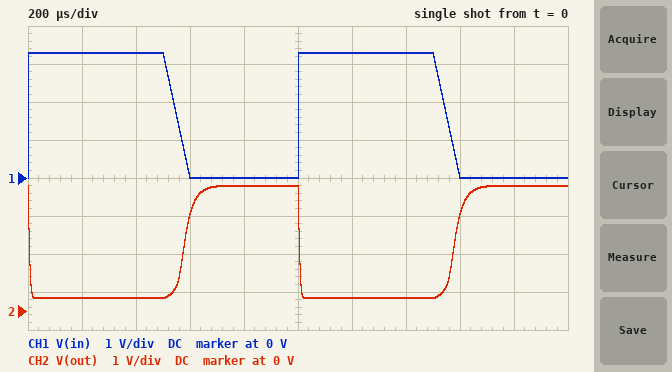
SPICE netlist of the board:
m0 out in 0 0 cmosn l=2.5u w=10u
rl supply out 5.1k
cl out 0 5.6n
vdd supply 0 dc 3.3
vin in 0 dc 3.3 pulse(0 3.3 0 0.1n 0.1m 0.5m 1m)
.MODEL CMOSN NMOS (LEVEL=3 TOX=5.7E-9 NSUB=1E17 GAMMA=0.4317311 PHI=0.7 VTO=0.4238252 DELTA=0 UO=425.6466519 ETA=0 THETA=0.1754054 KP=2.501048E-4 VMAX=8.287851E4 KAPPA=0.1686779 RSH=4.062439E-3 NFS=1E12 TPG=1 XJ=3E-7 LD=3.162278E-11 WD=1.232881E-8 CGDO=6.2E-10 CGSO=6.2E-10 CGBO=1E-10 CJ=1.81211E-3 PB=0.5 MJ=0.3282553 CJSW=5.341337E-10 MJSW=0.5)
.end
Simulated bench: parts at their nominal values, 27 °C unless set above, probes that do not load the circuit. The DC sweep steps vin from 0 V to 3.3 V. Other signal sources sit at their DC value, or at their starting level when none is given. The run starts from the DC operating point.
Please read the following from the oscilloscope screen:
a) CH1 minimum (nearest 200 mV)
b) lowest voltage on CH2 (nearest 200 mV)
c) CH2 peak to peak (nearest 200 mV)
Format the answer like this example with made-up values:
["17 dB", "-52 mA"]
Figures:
["0 V", "400 mV", "3.0 V"]
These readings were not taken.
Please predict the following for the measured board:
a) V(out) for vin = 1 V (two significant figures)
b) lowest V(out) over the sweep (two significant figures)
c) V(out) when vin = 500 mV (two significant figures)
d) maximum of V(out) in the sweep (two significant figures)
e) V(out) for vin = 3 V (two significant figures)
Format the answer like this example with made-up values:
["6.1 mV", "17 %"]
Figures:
["2.6 V", "340 mV", "3.3 V", "3.3 V", "370 mV"]
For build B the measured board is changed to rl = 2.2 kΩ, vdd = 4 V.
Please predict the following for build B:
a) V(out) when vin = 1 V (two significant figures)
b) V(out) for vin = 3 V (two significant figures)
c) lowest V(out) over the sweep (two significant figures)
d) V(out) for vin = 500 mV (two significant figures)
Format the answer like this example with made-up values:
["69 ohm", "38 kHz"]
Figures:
["3.7 V", "1.1 V", "1.0 V", "4.0 V"]
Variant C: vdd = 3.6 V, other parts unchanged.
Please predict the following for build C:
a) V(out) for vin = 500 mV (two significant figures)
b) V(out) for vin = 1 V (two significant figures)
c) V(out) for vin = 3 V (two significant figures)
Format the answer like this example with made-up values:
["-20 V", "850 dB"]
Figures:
["3.6 V", "2.9 V", "410 mV"]
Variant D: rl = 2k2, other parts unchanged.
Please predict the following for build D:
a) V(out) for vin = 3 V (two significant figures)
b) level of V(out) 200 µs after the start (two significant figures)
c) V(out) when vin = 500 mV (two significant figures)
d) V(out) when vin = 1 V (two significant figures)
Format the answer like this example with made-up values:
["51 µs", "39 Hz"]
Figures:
["860 mV", "780 mV", "3.3 V", "3.0 V"]
